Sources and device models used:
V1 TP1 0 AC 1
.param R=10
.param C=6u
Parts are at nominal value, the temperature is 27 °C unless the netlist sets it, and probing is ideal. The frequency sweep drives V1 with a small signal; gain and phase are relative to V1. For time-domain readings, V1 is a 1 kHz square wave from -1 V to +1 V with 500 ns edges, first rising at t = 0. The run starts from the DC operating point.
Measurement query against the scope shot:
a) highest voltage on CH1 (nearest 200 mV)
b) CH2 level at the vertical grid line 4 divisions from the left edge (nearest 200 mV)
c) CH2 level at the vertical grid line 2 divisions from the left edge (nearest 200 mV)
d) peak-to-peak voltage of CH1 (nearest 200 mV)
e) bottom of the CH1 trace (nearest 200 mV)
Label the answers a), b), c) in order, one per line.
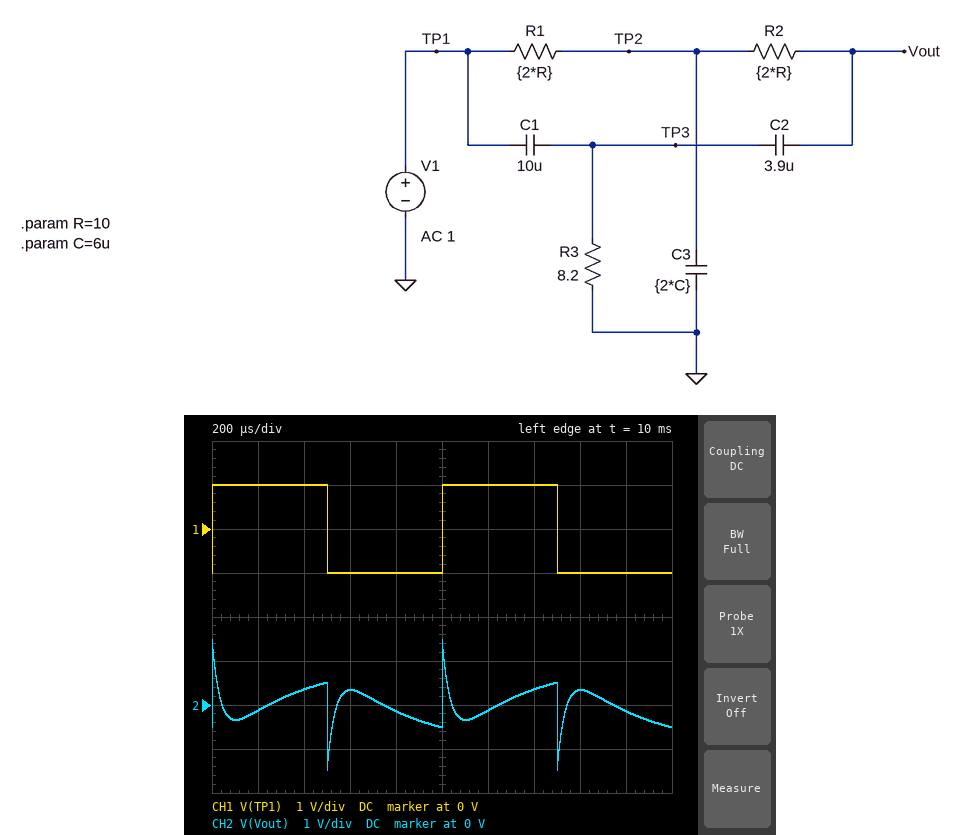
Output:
a) 1.0 V
b) -200 mV
c) 400 mV
d) 2.0 V
e) -1.0 V
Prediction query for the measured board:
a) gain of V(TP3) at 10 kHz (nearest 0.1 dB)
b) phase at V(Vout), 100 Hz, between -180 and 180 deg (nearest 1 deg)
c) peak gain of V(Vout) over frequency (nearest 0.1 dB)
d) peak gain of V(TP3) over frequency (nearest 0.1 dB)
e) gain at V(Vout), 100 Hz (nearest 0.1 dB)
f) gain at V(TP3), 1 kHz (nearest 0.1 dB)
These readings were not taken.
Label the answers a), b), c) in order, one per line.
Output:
a) -0.5 dB
b) -14 deg
c) 0 dB
d) 0 dB
e) -0.3 dB
f) -7.4 dB
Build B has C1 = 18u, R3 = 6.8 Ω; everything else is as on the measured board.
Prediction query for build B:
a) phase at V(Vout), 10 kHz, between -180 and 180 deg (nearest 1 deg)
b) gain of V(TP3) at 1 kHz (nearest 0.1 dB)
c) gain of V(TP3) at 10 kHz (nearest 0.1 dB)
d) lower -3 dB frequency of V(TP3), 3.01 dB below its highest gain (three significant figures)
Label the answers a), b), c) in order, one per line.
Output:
a) 21 deg
b) -4.9 dB
c) -0.2 dB
d) 1.69 kHz
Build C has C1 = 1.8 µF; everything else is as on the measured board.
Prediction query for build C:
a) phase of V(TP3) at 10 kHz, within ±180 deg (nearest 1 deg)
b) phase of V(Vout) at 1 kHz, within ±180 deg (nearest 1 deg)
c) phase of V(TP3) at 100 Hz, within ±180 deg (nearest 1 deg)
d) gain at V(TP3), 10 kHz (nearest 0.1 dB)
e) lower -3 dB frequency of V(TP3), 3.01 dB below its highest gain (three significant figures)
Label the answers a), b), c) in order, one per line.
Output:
a) 53 deg
b) -82 deg
c) 79 deg
d) -5.6 dB
e) 16.2 kHz
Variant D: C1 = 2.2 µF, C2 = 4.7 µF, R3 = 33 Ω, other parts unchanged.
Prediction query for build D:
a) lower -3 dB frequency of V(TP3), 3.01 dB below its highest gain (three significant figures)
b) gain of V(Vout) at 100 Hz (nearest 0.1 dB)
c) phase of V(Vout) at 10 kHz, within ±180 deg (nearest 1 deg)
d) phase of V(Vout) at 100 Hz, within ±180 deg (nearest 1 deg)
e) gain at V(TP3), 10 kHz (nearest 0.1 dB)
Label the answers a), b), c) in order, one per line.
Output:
a) 7.36 kHz
b) -0.4 dB
c) 37 deg
d) -15 deg
e) -1.9 dB
